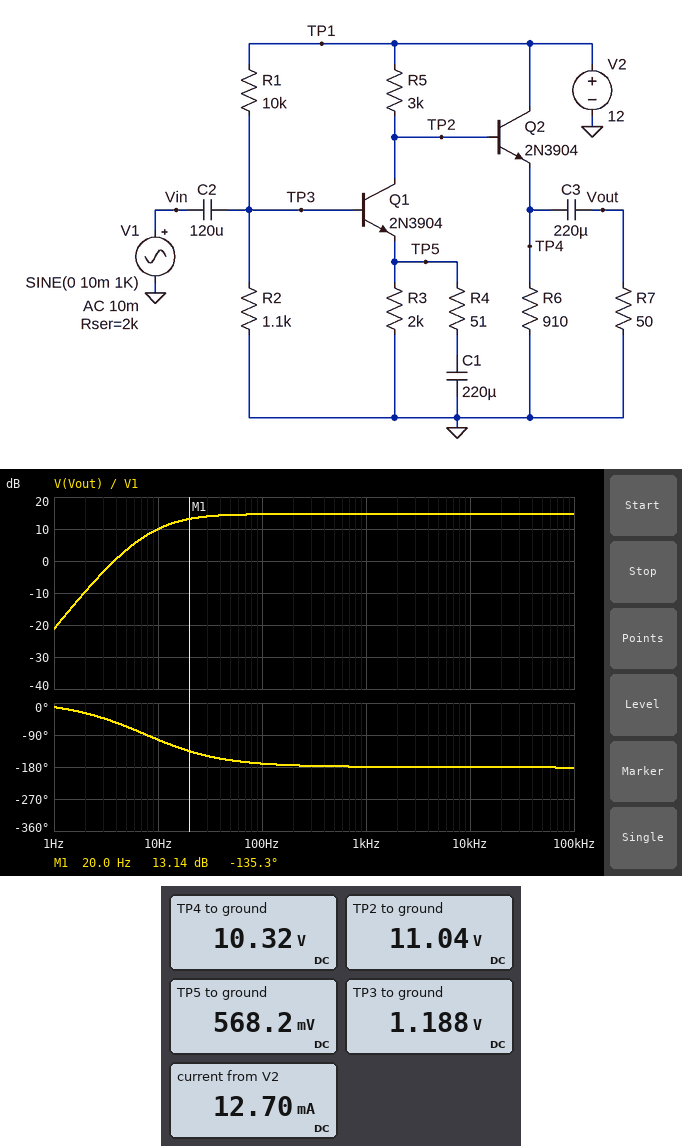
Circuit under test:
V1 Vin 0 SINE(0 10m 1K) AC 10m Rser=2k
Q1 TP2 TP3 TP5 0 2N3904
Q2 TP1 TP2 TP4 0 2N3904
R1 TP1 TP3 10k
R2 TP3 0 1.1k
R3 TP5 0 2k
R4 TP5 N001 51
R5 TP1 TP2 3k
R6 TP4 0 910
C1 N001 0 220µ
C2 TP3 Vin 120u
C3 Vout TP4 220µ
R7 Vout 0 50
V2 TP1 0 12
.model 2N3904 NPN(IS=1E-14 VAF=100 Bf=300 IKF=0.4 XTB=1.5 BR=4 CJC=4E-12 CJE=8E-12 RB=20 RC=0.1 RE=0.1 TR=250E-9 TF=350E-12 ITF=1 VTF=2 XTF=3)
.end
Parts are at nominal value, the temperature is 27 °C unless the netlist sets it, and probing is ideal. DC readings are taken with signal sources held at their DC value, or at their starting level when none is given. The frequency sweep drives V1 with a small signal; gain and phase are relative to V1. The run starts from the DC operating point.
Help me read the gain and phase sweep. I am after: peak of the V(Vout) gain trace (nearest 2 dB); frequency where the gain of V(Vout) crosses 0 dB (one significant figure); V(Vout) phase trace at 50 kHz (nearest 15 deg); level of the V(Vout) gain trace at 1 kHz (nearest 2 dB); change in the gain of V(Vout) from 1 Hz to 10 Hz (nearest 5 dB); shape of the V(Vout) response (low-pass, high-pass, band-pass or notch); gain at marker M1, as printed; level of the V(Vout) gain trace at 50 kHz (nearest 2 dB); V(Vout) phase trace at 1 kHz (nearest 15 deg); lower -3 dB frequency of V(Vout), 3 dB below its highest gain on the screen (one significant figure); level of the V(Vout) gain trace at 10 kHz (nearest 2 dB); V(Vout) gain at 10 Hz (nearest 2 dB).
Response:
14 dB
4 Hz
-180 deg
14 dB
30 dB
high-pass
13.14 dB
14 dB
-180 deg
10 Hz
14 dB
10 dB
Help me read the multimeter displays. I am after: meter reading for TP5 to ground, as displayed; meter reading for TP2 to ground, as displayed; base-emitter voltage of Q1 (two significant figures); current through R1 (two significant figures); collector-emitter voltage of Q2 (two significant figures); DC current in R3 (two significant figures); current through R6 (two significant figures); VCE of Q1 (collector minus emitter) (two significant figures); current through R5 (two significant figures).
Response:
568.2 mV
11.04 V
620 mV
1.1 mA
1.7 V
280 µA
11 mA
10 V
320 µA
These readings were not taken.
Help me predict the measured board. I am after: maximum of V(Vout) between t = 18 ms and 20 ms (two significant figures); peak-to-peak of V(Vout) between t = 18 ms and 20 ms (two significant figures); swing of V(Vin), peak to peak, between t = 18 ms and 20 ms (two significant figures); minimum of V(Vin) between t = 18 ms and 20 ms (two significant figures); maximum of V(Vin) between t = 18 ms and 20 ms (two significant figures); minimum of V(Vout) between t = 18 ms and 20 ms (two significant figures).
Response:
54 mV
110 mV
6.5 mV
-3.3 mV
3.3 mV
-55 mV
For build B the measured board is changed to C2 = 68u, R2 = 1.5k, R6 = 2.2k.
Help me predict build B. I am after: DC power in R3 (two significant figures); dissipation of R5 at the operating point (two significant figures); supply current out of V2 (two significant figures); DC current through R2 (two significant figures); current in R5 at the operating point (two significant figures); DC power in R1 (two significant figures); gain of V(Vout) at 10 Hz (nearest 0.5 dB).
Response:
430 µW
690 µW
6.0 mA
1.0 mA
480 µA
11 mW
13.0 dB
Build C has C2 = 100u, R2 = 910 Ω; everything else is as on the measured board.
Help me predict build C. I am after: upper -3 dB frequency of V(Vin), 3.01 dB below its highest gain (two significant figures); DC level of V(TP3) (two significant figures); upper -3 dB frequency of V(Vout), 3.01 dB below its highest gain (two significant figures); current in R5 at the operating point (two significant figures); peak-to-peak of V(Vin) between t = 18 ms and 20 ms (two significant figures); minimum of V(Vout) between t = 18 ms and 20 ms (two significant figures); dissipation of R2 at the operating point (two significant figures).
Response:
620 mHz
1.0 V
3.3 MHz
230 µA
5.8 mV
-38 mV
1.1 mW
